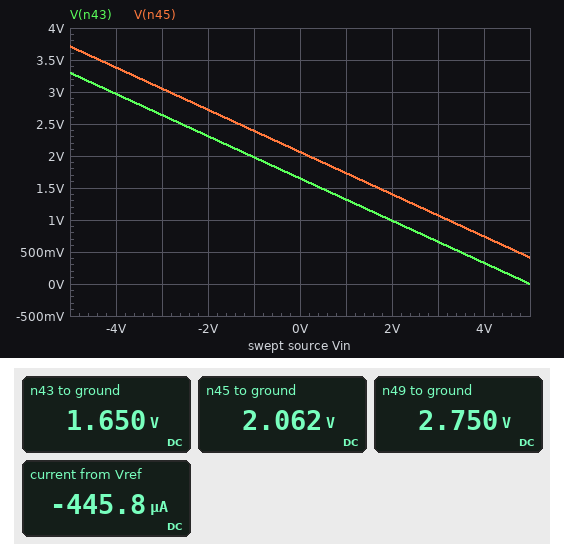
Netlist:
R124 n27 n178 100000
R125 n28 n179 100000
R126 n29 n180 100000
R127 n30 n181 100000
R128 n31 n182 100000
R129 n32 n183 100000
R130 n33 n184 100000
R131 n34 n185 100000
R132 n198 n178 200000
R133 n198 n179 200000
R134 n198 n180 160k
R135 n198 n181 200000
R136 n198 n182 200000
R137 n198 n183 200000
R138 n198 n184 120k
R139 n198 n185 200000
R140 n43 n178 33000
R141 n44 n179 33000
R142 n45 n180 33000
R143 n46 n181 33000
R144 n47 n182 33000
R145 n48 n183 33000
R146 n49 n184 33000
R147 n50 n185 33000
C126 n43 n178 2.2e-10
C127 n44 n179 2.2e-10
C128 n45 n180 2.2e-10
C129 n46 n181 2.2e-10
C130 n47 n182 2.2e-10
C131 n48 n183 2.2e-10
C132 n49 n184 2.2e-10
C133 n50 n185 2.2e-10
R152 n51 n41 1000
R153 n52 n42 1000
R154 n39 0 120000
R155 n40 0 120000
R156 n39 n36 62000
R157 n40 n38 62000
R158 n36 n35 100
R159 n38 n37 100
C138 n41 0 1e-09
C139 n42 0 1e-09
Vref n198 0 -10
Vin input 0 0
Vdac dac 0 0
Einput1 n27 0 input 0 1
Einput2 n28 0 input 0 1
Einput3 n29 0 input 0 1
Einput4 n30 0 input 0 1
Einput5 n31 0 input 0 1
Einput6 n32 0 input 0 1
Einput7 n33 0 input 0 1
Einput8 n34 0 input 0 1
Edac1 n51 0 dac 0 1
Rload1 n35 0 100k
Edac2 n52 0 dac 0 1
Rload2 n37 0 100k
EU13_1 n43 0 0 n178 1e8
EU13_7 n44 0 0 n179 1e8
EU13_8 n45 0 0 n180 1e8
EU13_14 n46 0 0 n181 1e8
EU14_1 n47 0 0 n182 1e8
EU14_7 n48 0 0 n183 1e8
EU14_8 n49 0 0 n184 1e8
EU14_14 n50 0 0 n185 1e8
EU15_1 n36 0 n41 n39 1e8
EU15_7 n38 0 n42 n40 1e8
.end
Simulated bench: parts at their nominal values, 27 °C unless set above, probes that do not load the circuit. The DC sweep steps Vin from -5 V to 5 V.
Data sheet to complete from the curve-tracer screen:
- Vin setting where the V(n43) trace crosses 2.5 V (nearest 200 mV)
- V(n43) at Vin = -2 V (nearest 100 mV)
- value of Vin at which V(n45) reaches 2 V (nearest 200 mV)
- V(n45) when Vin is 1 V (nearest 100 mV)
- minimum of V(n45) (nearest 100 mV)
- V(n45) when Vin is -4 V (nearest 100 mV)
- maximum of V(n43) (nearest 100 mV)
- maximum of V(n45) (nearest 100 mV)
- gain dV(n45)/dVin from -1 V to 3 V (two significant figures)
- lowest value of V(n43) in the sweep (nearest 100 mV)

-2.6 V
2.3 V
200 mV
1.7 V
400 mV
3.4 V
3.3 V
3.7 V
-0.33 V/V
0 V
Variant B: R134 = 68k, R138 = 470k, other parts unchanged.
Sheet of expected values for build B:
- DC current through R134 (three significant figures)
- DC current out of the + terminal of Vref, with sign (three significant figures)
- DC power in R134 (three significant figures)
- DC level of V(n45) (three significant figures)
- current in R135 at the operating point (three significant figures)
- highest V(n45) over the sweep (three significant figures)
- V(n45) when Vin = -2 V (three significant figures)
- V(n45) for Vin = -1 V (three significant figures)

147 µA
-468 µA
1.47 mW
4.85 V
50.0 µA
6.50 V
5.51 V
5.18 V
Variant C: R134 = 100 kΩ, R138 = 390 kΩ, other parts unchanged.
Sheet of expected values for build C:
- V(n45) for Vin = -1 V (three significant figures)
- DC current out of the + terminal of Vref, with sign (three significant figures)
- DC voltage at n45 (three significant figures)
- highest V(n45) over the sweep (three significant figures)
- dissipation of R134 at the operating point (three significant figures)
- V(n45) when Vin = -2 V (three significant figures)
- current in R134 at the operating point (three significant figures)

3.63 V
-426 µA
3.30 V
4.95 V
1.00 mW
3.96 V
100 µA
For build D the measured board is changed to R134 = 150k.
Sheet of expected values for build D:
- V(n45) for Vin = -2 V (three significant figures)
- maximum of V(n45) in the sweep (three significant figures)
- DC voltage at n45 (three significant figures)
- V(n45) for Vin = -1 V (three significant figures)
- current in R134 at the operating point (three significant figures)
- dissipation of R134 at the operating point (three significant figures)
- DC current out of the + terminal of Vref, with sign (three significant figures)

2.86 V
3.85 V
2.20 V
2.53 V
66.7 µA
667 µW
-450 µA
